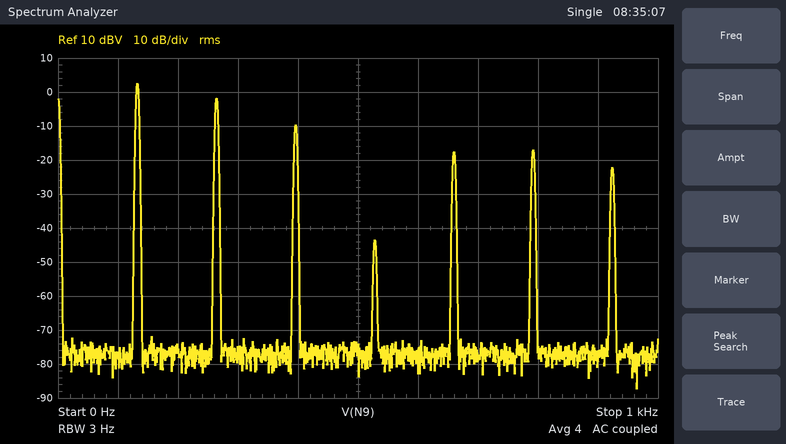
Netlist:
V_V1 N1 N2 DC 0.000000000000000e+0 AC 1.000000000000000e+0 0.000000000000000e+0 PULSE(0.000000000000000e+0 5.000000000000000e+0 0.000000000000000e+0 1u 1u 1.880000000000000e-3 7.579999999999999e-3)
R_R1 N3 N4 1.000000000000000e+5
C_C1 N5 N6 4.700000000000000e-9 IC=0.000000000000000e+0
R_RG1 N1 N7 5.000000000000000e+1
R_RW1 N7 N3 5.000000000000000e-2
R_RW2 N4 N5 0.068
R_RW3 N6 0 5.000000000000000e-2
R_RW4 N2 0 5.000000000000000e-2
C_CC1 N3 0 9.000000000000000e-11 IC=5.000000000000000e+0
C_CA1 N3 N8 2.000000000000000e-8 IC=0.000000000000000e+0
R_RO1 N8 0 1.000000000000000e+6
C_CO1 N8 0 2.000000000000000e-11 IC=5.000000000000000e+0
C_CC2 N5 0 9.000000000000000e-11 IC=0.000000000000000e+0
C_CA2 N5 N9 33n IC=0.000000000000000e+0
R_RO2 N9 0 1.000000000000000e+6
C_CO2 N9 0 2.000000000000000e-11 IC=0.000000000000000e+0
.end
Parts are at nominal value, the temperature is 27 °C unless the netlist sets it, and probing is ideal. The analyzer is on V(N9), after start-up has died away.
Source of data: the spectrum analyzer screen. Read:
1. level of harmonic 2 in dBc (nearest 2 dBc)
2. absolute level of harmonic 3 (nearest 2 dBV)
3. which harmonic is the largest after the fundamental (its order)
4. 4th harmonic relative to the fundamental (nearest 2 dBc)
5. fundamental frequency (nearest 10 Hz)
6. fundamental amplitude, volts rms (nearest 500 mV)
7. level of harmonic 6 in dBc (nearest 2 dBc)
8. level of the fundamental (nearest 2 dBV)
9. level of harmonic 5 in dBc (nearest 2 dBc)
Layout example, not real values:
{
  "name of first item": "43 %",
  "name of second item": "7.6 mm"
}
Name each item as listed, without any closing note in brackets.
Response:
{
  "level of harmonic 2 in dBc": "-4 dBc",
  "absolute level of harmonic 3": "-10 dBV",
  "which harmonic is the largest after the fundamental": "2",
  "4th harmonic relative to the fundamental": "-46 dBc",
  "fundamental frequency": "130 Hz",
  "fundamental amplitude, volts rms": "1.5 V",
  "level of harmonic 6 in dBc": "-20 dBc",
  "level of the fundamental": "2 dBV",
  "level of harmonic 5 in dBc": "-20 dBc"
}
